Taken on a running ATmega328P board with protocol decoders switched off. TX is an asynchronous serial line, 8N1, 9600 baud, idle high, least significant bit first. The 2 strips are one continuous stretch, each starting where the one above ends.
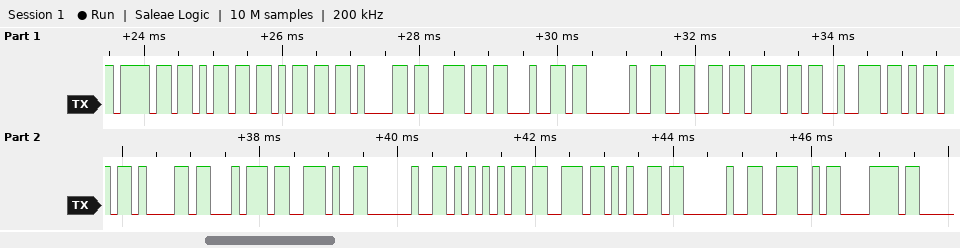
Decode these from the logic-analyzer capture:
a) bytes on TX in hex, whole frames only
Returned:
0x6F 0x6D 0x6D 0x61 0x6E 0x64 0x20 0x66 0x6F 0x72 0x6D 0x61 0x74 0x2E 0x20 0x55 0x73 0x65 0x20 0x4E 0x78
